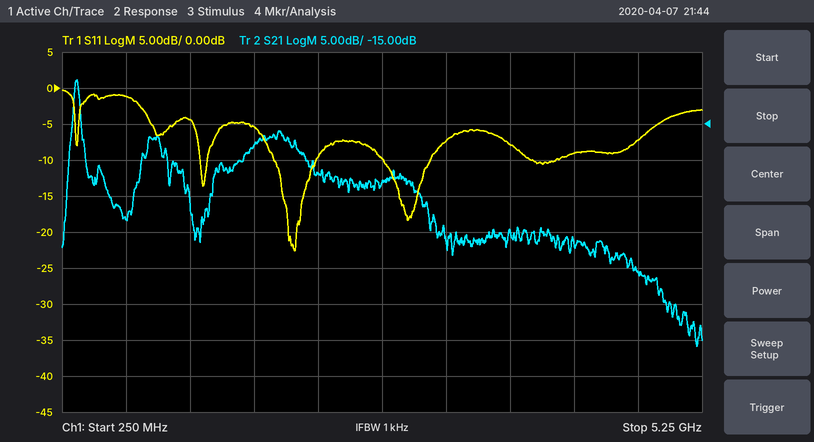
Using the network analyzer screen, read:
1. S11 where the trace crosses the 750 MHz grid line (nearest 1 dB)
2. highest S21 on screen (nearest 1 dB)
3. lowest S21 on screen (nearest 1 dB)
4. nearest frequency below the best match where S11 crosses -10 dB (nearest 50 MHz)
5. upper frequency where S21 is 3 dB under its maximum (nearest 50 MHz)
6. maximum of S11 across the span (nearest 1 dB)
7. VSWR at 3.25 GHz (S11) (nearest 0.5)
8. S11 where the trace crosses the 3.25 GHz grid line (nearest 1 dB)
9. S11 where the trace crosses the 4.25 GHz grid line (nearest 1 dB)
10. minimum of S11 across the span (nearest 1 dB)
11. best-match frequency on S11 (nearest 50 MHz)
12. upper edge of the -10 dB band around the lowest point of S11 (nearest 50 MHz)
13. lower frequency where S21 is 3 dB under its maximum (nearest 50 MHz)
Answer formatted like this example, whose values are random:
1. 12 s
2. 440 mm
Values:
1. -1 dB
2. -9 dB
3. -46 dB
4. 1.90 GHz
5. 400 MHz
6. 0 dB
7. 2.5
8. -7 dB
9. -9 dB
10. -23 dB
11. 2.05 GHz
12. 2.25 GHz
13. 350 MHz
